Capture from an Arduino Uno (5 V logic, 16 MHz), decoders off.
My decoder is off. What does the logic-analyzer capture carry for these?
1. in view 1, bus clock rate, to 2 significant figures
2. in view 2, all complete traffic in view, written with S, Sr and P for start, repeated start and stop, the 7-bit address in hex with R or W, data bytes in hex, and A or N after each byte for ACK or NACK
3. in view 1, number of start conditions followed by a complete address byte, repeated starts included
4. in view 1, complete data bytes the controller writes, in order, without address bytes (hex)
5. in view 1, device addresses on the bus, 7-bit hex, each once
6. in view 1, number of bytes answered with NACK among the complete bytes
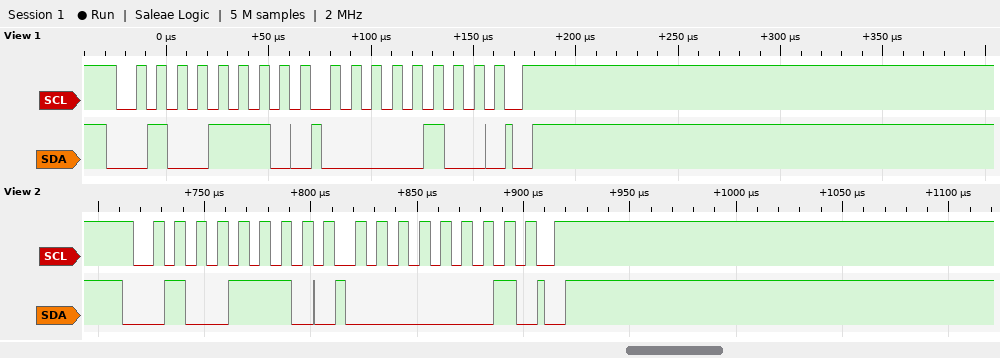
100 kHz
S 27W A 01 A P
1
04
0x27
0
